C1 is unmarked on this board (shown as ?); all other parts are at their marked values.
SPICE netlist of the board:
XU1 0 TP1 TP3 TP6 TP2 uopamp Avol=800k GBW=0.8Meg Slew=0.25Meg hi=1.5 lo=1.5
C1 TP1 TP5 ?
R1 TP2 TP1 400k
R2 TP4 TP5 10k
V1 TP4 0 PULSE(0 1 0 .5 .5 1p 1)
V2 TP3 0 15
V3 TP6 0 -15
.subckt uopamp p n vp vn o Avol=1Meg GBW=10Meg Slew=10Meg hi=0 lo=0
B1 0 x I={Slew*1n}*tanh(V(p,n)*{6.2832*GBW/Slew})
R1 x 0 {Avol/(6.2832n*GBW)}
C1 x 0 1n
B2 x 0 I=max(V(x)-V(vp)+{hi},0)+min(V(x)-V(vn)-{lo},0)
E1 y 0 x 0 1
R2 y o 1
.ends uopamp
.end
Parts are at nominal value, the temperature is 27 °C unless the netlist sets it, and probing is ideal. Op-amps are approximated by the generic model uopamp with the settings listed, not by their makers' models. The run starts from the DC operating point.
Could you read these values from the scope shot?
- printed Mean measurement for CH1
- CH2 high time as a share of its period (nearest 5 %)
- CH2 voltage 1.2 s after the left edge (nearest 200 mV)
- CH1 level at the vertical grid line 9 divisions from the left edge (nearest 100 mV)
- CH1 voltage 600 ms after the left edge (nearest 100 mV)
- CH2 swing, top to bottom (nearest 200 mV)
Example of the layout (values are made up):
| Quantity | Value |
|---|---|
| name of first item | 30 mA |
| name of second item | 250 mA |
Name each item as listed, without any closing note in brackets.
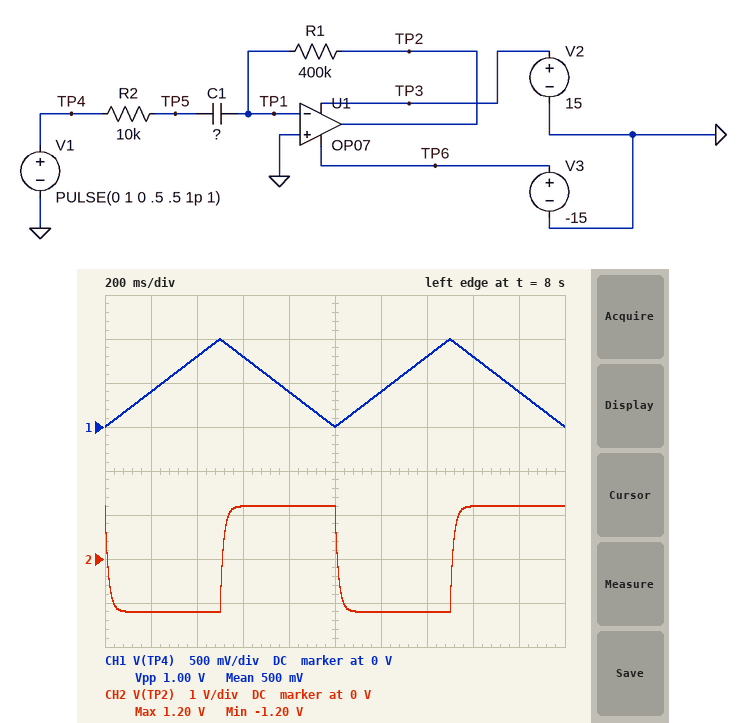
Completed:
| Quantity | Value |
|---|---|
| printed Mean measurement for CH1 | 500 mV |
| CH2 high time as a share of its period | 50 % |
| CH2 voltage 1.2 s after the left edge | -1.2 V |
| CH1 level at the vertical grid line 9 divisions from the left edge | 400 mV |
| CH1 voltage 600 ms after the left edge | 800 mV |
| CH2 swing, top to bottom | 2.4 V |
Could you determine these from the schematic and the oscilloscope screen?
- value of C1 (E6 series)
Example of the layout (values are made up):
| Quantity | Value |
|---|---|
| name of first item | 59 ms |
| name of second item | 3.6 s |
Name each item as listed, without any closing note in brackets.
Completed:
| Quantity | Value |
|---|---|
| value of C1 | 1.5 µF |
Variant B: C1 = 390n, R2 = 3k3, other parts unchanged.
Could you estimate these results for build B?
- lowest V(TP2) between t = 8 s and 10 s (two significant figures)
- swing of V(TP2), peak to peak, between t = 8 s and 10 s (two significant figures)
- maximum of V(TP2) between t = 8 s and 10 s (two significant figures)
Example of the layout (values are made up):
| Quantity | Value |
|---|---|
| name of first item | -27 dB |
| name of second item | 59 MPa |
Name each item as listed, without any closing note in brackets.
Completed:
| Quantity | Value |
|---|---|
| lowest V(TP2) between t = 8 s and 10 s | -310 mV |
| swing of V(TP2), peak to peak, between t = 8 s and 10 s | 620 mV |
| maximum of V(TP2) between t = 8 s and 10 s | 310 mV |
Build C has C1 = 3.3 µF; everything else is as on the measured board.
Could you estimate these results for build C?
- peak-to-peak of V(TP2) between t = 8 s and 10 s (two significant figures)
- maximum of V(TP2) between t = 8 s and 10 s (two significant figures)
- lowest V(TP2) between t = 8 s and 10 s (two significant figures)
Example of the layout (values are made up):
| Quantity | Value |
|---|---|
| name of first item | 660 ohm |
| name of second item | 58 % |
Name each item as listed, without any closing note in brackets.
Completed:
| Quantity | Value |
|---|---|
| peak-to-peak of V(TP2) between t = 8 s and 10 s | 5.3 V |
| maximum of V(TP2) between t = 8 s and 10 s | 2.6 V |
| lowest V(TP2) between t = 8 s and 10 s | -2.6 V |
